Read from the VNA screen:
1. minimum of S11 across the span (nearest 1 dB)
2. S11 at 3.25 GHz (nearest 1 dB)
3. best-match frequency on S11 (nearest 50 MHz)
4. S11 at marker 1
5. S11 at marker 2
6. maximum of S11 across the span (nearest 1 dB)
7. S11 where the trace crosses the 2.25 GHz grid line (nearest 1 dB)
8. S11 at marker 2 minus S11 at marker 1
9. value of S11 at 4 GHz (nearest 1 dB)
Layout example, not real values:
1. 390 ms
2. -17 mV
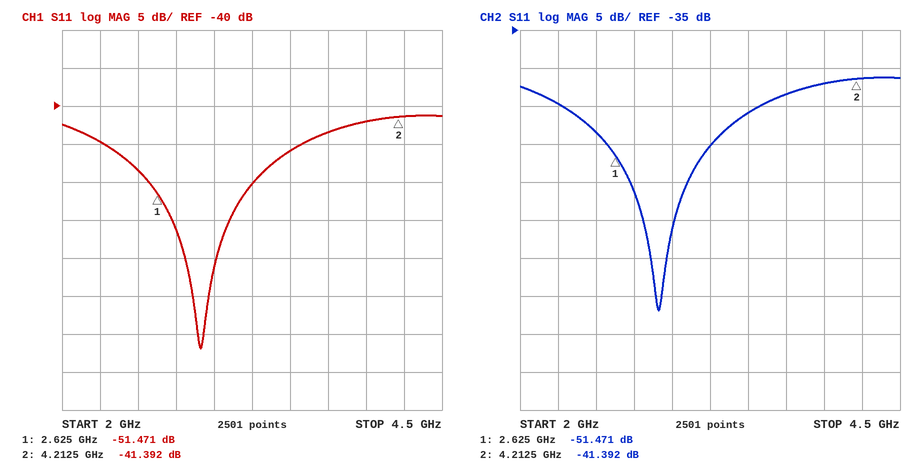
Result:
1. -72 dB
2. -50 dB
3. 2.90 GHz
4. -51.471 dB
5. -41.392 dB
6. -41 dB
7. -45 dB
8. 10.079 dB
9. -42 dB
